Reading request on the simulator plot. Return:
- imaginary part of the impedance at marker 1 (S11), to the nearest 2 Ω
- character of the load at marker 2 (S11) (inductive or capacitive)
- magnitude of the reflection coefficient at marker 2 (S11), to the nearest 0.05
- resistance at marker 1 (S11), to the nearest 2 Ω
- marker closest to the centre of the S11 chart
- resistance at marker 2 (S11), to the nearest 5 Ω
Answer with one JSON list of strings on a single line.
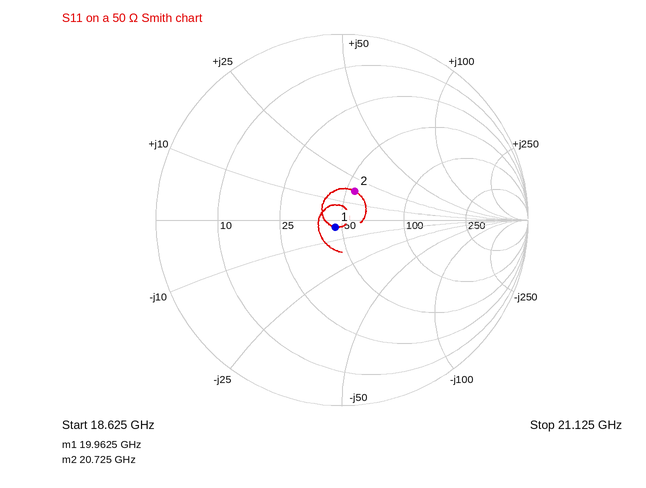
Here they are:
["-4 Ω", "inductive", "0.15", "46 Ω", "marker 1", "55 Ω"]
